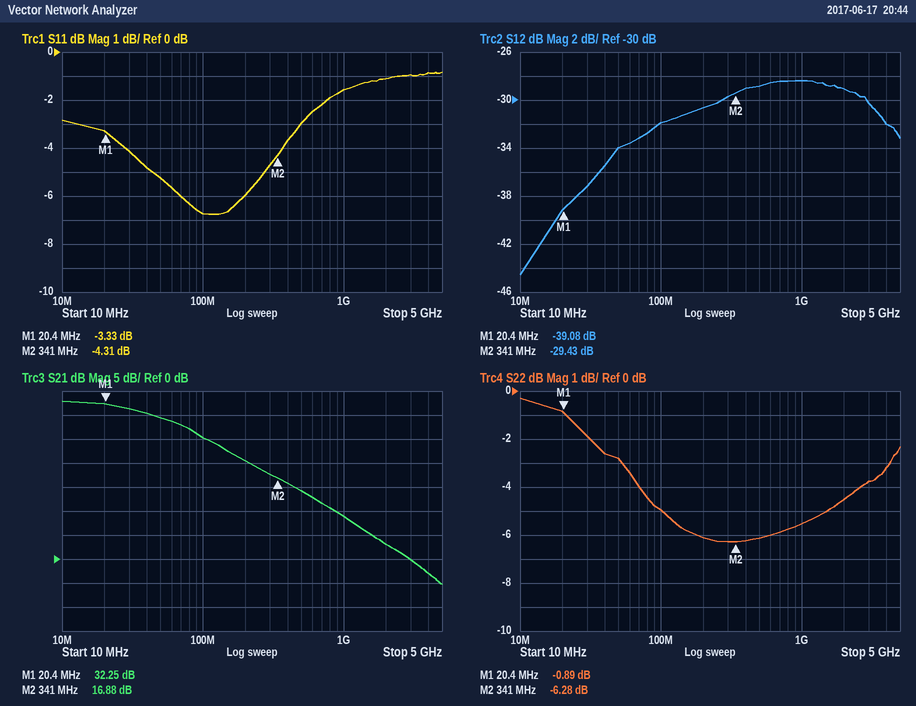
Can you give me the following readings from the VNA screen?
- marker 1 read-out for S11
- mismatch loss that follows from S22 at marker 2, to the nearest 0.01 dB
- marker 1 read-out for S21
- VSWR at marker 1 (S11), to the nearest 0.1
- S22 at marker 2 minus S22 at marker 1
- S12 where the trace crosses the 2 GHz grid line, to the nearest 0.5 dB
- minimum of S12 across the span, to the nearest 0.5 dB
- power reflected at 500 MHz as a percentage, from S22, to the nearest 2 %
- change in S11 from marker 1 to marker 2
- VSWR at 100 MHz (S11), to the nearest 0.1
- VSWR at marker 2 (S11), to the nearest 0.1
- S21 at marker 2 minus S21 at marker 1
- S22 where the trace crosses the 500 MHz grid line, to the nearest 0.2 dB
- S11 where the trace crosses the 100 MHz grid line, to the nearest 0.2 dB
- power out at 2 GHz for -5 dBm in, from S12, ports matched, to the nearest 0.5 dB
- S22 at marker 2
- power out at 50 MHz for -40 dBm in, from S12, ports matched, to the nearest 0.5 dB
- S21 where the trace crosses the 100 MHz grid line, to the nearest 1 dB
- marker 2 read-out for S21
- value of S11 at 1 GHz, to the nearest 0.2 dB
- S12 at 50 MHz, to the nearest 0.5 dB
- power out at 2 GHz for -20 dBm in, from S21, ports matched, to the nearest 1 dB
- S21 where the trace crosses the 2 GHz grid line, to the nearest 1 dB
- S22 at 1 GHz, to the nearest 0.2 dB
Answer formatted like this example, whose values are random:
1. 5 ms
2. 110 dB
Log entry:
1. -3.33 dB
2. 1.17 dB
3. 32.25 dB
4. 5.3
5. -5.39 dB
6. -29.0 dB
7. -44.5 dB
8. 24 %
9. -0.98 dB
10. 2.7
11. 4.1
12. -15.37 dB
13. -6.2 dB
14. -6.8 dB
15. -34.0 dBm
16. -6.28 dB
17. -74.0 dBm
18. 25 dB
19. 16.88 dB
20. -1.6 dB
21. -34.0 dB
22. -17 dBm
23. 3 dB
24. -5.6 dB
